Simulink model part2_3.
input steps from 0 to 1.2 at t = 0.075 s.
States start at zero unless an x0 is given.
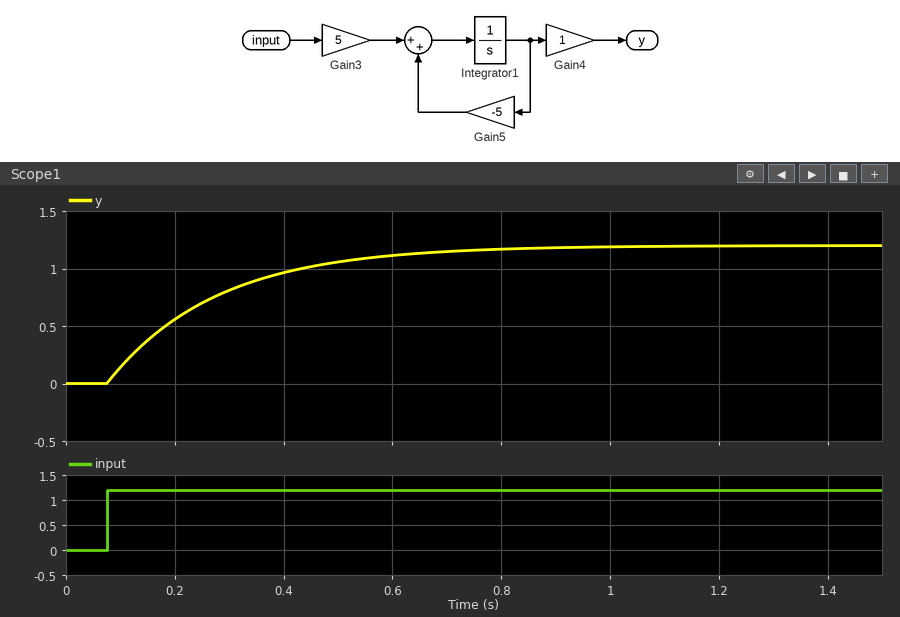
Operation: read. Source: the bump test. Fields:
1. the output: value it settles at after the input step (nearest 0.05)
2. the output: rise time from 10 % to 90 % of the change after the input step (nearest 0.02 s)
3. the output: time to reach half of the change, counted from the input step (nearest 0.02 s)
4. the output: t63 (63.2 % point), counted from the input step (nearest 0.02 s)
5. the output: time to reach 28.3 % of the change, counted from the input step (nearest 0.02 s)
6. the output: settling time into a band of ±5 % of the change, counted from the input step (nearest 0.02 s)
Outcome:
1.20
0.44 s
0.14 s
0.20 s
0.06 s
0.60 s
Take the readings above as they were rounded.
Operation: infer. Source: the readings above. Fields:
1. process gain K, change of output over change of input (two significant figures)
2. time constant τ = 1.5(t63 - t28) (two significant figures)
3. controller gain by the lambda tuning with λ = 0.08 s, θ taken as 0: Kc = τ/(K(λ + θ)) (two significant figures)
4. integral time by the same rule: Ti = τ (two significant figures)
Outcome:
1.0
0.21 s
2.6
0.21 s
